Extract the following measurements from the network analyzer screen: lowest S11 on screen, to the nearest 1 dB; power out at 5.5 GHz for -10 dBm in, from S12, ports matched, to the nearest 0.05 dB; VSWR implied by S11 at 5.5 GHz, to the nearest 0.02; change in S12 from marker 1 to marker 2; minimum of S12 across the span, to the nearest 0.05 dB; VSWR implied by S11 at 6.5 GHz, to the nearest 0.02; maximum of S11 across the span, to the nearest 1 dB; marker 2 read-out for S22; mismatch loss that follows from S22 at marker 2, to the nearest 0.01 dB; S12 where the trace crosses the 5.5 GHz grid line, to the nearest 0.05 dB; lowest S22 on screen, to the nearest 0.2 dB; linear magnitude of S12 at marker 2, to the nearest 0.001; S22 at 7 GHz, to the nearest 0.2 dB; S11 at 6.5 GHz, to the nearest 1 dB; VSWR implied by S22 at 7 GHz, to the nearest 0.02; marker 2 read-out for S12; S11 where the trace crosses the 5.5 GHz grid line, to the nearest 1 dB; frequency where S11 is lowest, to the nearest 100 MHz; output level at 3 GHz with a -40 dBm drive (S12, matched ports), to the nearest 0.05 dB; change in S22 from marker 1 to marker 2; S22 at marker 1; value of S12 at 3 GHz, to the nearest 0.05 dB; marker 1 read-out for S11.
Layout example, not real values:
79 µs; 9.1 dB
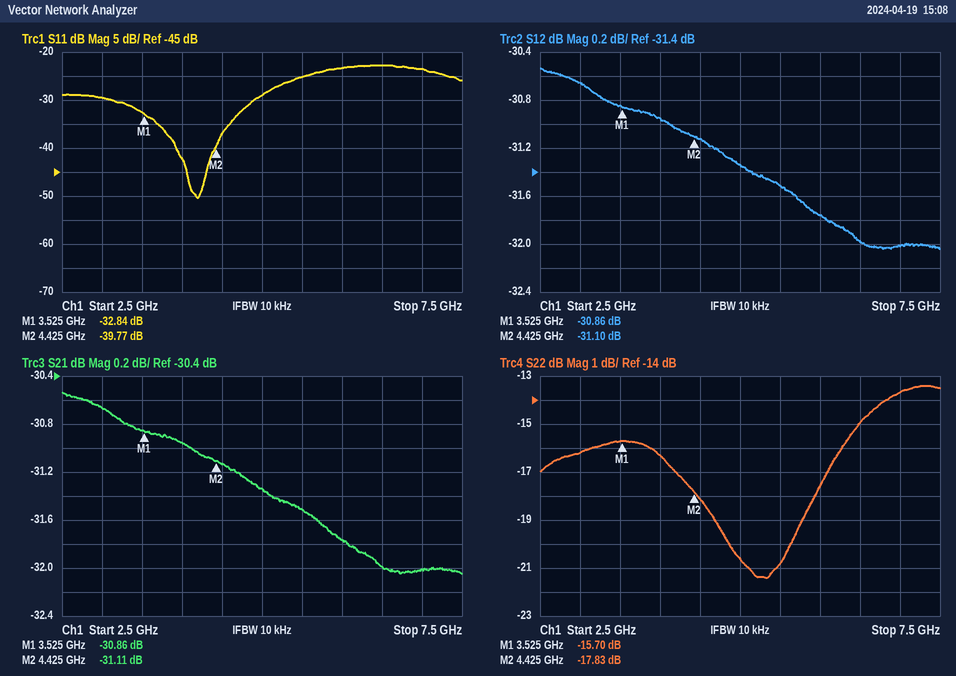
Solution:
-50 dB; -41.50 dBm; 1.12; -0.24 dB; -32.05 dB; 1.16; -23 dB; -17.83 dB; 0.07 dB; -31.50 dB; -21.4 dB; 0.028; -13.6 dB; -23 dB; 1.52; -31.10 dB; -25 dB; 4.2 GHz; -70.65 dBm; -2.13 dB; -15.70 dB; -30.65 dB; -32.84 dB
